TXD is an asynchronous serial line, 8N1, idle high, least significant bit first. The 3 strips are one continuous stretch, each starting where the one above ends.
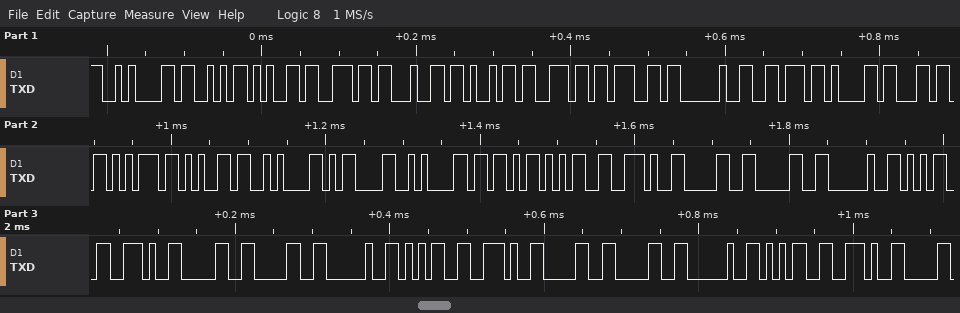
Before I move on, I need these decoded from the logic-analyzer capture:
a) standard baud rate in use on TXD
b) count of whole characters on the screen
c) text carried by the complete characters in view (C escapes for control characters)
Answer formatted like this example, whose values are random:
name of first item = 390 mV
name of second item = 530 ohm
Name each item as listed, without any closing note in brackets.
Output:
standard baud rate in use on TXD = 115200 baud
count of whole characters on the screen = 35
text carried by the complete characters in view = "\nSending value\n\r\n[5.00 5.00 5.00 5."
